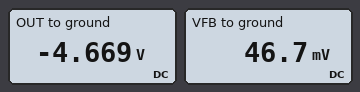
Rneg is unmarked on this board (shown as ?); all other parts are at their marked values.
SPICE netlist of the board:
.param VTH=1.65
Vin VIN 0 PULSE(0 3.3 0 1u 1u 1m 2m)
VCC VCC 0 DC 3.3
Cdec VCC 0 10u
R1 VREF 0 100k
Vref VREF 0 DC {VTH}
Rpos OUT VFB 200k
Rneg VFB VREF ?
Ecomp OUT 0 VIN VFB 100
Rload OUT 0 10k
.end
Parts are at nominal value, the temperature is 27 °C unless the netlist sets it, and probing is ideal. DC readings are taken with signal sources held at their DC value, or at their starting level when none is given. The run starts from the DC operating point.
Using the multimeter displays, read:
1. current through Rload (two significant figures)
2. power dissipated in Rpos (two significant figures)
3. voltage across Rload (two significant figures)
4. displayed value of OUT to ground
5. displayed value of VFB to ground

470 µA
110 µW
4.7 V
-4.669 V
46.7 mV
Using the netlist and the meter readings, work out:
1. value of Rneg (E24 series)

68 kΩ
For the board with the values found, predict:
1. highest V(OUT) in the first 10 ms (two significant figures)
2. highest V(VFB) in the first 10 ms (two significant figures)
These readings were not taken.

7.8 V
3.2 V
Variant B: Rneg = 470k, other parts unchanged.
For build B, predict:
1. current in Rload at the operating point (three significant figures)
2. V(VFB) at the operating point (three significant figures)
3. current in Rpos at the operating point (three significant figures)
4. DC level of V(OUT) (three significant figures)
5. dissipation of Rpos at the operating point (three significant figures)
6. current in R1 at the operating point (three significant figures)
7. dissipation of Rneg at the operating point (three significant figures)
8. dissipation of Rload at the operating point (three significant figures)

69.2 µA
6.92 mV
3.50 µA
-692 mV
2.44 µW
16.5 µA
5.74 µW
47.9 µW
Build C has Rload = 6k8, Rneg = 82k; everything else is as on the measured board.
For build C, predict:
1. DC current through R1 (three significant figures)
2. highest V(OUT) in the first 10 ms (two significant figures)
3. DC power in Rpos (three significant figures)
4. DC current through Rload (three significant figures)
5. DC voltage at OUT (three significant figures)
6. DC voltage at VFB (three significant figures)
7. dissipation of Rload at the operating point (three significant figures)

16.5 µA
7.1 V
77.2 µW
572 µA
-3.89 V
38.9 mV
2.23 mW
